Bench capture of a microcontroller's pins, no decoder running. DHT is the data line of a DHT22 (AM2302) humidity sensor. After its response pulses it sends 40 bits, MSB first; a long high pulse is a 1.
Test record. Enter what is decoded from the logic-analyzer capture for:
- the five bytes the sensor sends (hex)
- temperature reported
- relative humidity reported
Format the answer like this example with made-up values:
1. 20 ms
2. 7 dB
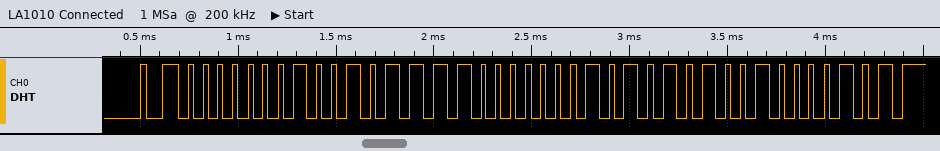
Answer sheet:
1. 01 2F 01 54 85
2. 34.0 °C
3. 30.3 %
